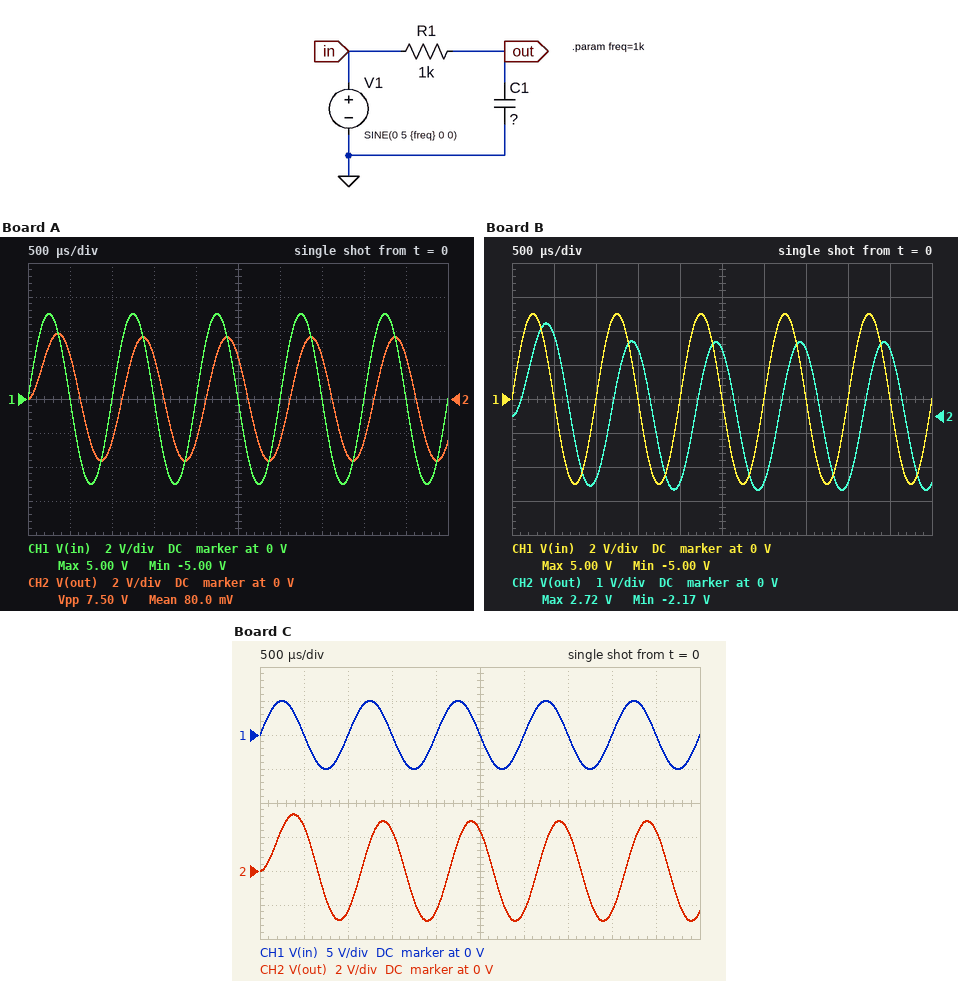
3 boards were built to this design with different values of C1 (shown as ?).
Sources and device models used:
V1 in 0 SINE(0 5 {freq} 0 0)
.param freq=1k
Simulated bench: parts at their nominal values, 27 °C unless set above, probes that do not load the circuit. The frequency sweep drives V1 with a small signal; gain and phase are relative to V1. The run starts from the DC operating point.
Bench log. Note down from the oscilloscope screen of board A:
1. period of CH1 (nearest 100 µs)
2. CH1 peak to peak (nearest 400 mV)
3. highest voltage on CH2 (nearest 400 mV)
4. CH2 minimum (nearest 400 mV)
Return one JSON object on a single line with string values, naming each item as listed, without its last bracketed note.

{"period of CH1": "1.0 ms", "CH1 peak to peak": "10.0 V", "highest voltage on CH2": "4.0 V", "CH2 minimum": "-3.6 V"}
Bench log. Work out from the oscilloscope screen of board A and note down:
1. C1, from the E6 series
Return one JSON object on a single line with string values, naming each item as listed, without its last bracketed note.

{"C1, from the E6 series": "150 nF"}
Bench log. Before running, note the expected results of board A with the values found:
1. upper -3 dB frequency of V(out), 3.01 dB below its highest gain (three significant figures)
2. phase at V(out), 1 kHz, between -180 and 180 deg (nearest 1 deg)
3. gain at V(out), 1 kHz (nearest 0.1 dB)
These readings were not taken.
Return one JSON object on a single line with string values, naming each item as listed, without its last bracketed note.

{"upper -3 dB frequency of V(out), 3.01 dB below its highest gain": "1.06 kHz", "phase at V(out), 1 kHz, between -180 and 180 deg": "-43 deg", "gain at V(out), 1 kHz": "-2.8 dB"}
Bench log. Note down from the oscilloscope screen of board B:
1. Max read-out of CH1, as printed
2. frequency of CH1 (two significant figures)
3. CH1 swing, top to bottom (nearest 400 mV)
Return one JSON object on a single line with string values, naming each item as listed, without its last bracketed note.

{"Max read-out of CH1, as printed": "5.00 V", "frequency of CH1": "1.0 kHz", "CH1 swing, top to bottom": "10.0 V"}
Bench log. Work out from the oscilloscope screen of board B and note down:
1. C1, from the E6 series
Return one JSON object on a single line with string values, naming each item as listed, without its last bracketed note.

{"C1, from the E6 series": "330 nF"}
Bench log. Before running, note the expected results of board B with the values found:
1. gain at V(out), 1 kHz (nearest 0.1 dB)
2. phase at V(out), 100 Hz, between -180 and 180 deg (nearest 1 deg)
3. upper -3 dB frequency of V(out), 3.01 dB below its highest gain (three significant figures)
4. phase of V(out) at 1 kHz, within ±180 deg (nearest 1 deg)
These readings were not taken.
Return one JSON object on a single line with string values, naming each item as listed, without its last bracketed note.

{"gain at V(out), 1 kHz": "-7.2 dB", "phase at V(out), 100 Hz, between -180 and 180 deg": "-12 deg", "upper -3 dB frequency of V(out), 3.01 dB below its highest gain": "482 Hz", "phase of V(out) at 1 kHz, within ±180 deg": "-64 deg"}
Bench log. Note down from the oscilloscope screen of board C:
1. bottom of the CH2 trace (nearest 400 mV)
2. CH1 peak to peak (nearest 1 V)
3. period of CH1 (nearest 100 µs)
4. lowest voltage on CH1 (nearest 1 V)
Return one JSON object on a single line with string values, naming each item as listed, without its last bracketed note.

{"bottom of the CH2 trace": "-2.8 V", "CH1 peak to peak": "10 V", "period of CH1": "1.0 ms", "lowest voltage on CH1": "-5 V"}
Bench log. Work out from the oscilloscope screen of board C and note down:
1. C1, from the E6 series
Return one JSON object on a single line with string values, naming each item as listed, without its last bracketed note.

{"C1, from the E6 series": "220 nF"}
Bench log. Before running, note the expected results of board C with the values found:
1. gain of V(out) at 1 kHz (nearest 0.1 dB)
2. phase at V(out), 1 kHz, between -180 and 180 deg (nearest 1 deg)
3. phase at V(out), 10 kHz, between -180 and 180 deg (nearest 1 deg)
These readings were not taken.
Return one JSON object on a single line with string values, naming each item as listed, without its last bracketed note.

{"gain of V(out) at 1 kHz": "-4.6 dB", "phase at V(out), 1 kHz, between -180 and 180 deg": "-54 deg", "phase at V(out), 10 kHz, between -180 and 180 deg": "-86 deg"}
